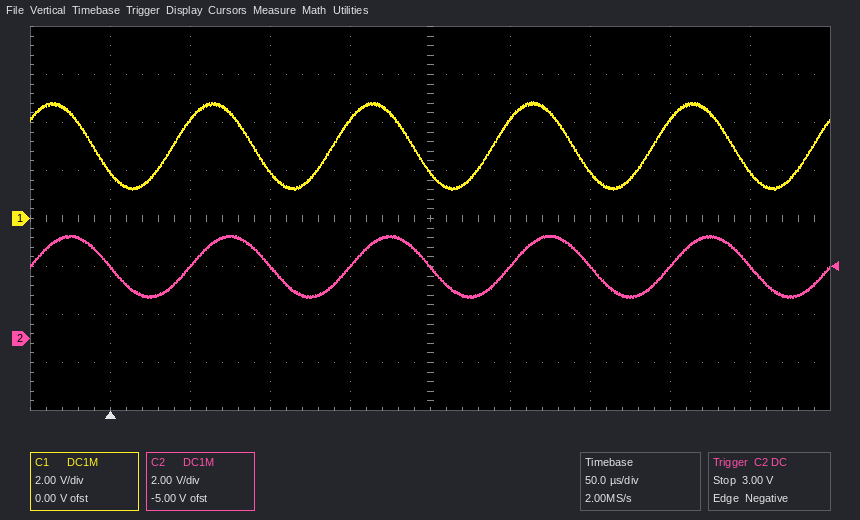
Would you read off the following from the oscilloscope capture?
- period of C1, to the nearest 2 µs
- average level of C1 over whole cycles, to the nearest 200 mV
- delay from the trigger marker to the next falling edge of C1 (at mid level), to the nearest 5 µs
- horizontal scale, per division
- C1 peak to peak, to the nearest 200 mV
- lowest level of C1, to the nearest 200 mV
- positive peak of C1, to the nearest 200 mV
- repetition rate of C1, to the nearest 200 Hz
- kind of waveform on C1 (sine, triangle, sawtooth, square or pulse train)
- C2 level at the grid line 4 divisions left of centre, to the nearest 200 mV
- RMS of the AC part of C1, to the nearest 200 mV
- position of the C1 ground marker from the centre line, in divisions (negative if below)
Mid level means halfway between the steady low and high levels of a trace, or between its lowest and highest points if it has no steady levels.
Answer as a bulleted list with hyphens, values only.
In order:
- 100 µs
- 3.0 V
- 90 µs
- 50 µs
- 3.6 V
- 1.2 V
- 4.8 V
- 10.0 kHz
- sine
- 3.0 V
- 1.2 V
- 0.0 div
